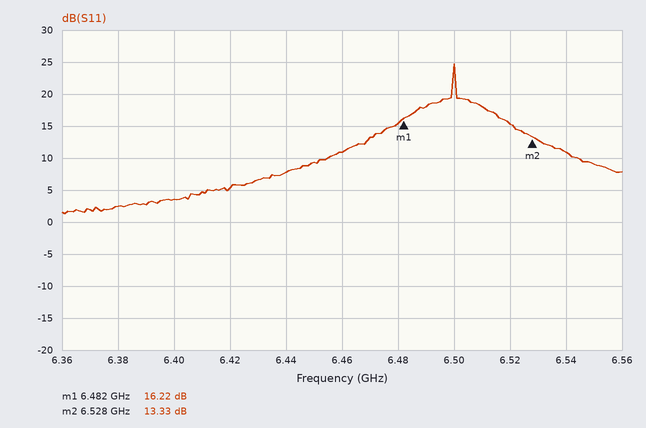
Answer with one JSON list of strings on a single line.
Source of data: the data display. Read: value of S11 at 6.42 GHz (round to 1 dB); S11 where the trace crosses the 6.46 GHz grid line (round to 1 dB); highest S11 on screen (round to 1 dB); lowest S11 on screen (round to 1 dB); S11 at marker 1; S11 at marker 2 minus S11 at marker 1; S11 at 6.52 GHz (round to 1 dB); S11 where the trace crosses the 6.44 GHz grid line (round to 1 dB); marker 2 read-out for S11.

["5 dB", "11 dB", "25 dB", "1 dB", "16.22 dB", "-2.89 dB", "15 dB", "8 dB", "13.33 dB"]
